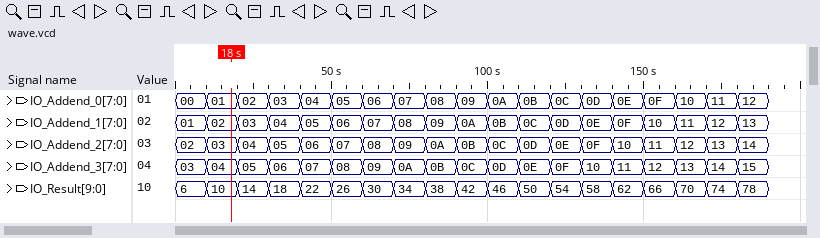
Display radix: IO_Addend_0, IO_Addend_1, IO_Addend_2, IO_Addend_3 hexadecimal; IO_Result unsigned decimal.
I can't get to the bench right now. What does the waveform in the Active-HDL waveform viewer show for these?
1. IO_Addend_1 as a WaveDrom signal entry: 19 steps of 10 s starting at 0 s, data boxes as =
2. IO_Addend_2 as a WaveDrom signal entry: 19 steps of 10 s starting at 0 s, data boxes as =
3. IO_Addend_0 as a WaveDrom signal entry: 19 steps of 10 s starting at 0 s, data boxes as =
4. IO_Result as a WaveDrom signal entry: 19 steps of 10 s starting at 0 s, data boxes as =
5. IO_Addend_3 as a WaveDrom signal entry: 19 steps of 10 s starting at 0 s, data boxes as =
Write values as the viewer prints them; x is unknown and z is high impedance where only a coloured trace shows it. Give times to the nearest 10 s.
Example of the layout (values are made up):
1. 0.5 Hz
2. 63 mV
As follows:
1. {name: 'IO_Addend_1', wave: '===================', data: '01 02 03 04 05 06 07 08 09 0A 0B 0C 0D 0E 0F 10 11 12 13'}
2. {name: 'IO_Addend_2', wave: '===================', data: '02 03 04 05 06 07 08 09 0A 0B 0C 0D 0E 0F 10 11 12 13 14'}
3. {name: 'IO_Addend_0', wave: '===================', data: '00 01 02 03 04 05 06 07 08 09 0A 0B 0C 0D 0E 0F 10 11 12'}
4. {name: 'IO_Result', wave: '===================', data: '6 10 14 18 22 26 30 34 38 42 46 50 54 58 62 66 70 74 78'}
5. {name: 'IO_Addend_3', wave: '===================', data: '03 04 05 06 07 08 09 0A 0B 0C 0D 0E 0F 10 11 12 13 14 15'}
